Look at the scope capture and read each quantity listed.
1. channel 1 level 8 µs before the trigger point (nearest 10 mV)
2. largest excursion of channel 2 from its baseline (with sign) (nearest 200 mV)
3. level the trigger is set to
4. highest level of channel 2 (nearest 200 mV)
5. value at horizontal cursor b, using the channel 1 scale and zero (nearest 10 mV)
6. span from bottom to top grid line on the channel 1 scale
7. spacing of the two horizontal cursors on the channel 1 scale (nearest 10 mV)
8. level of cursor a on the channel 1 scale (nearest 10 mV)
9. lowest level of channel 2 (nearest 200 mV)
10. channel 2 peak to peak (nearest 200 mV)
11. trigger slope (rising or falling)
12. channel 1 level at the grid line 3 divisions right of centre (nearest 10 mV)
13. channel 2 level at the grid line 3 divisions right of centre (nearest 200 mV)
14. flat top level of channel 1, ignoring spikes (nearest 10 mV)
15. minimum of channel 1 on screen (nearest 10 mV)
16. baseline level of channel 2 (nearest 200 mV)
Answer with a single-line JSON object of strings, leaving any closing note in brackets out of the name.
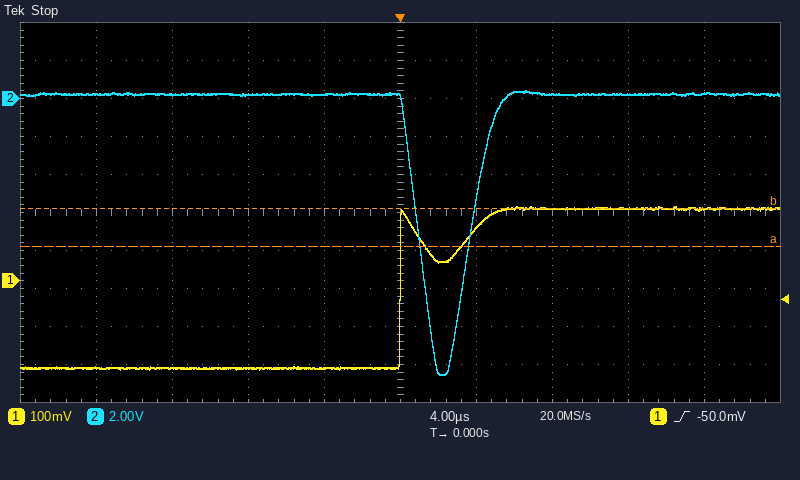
{"channel 1 level 8 µs before the trigger point": "-230 mV", "largest excursion of channel 2 from its baseline (with sign)": "-14.8 V", "level the trigger is set to": "-50.0 mV", "highest level of channel 2": "400 mV", "value at horizontal cursor b, using the channel 1 scale and zero": "190 mV", "span from bottom to top grid line on the channel 1 scale": "1 V", "spacing of the two horizontal cursors on the channel 1 scale": "100 mV", "level of cursor a on the channel 1 scale": "90 mV", "lowest level of channel 2": "-14.6 V", "channel 2 peak to peak": "15.0 V", "trigger slope": "rising", "channel 1 level at the grid line 3 divisions right of centre": "190 mV", "channel 2 level at the grid line 3 divisions right of centre": "200 mV", "flat top level of channel 1, ignoring spikes": "190 mV", "minimum of channel 1 on screen": "-230 mV", "baseline level of channel 2": "200 mV"}
